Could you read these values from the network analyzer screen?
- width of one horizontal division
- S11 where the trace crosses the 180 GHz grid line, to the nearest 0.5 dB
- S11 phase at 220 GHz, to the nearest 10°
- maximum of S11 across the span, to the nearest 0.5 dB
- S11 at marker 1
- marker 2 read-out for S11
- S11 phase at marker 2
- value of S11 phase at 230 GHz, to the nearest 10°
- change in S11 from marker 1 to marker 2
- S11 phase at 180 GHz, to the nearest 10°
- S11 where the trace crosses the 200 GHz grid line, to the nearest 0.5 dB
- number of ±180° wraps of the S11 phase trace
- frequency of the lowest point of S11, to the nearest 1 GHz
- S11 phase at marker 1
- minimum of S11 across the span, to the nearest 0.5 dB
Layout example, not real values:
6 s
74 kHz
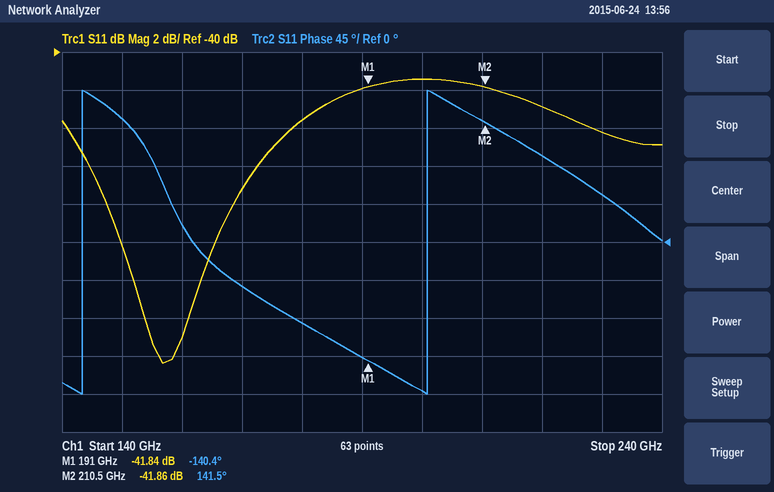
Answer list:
10 GHz
-43.5 dB
100°
-41.5 dB
-41.84 dB
-41.86 dB
141.5°
60°
-0.02 dB
-100°
-41.5 dB
2
157 GHz
-140.4°
-56.5 dB
